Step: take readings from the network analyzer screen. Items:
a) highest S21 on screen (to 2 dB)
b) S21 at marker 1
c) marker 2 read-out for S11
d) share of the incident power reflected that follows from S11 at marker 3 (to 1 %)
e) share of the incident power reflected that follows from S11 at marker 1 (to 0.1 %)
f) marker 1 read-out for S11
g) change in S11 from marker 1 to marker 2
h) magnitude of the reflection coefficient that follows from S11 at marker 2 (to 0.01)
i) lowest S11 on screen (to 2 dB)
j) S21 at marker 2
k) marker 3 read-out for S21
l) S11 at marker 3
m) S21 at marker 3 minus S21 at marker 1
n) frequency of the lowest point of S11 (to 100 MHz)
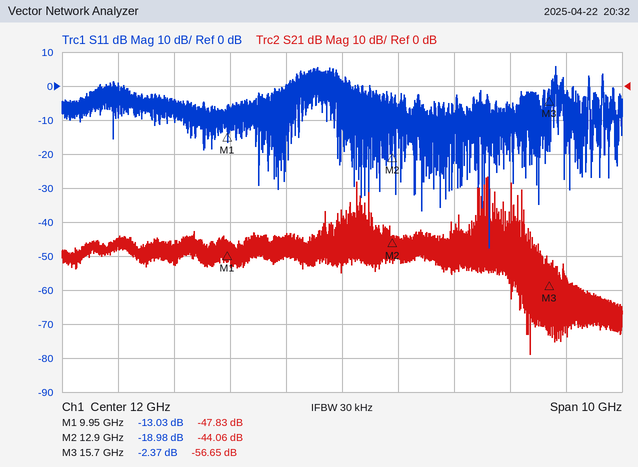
-26 dB
-47.83 dB
-18.98 dB
58 %
5.0 %
-13.03 dB
-5.95 dB
0.11
-48 dB
-44.06 dB
-56.65 dB
-2.37 dB
-8.82 dB
14.6 GHz
